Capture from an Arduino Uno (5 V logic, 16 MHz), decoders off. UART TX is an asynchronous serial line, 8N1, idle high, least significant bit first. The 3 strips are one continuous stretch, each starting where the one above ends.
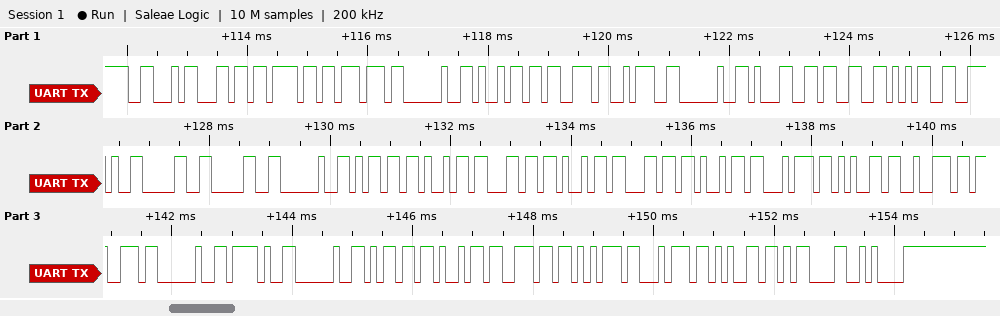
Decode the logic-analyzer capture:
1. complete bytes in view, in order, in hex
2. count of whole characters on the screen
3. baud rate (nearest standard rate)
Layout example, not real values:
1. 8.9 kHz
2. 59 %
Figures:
1. 46 6C 6F 77 20 69 73 3A 20 31 33 35 2E 30 30 20 6D 69 6C 69 6C 69 74 65 72 73 20 2F 20 6D 69 6E 75 74 65 0D 0A
2. 37
3. 9600 baud
